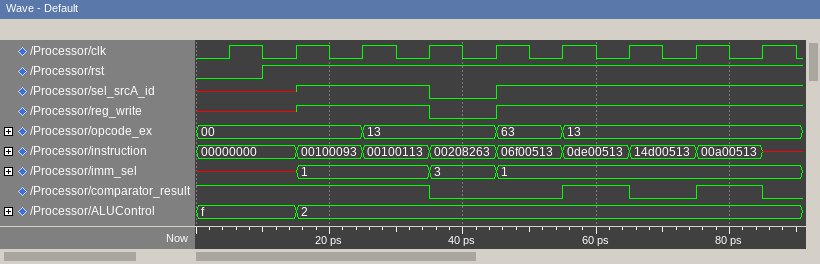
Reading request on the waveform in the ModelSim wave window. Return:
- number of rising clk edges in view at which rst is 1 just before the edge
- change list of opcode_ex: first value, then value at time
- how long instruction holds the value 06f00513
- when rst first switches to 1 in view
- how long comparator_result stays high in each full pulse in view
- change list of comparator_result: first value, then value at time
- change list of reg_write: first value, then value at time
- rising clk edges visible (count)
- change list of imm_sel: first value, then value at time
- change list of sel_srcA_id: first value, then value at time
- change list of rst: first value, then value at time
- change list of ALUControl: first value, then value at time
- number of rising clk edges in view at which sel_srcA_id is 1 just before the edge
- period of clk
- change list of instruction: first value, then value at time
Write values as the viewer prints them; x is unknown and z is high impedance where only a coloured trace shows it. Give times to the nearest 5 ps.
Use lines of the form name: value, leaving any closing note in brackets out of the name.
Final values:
number of rising clk edges in view at which rst is 1 just before the edge: 8
change list of opcode_ex: first value, then value at time: 00, 13 at 25 ps, 63 at 45 ps, 13 at 55 ps
how long instruction holds the value 06f00513: 10 ps
when rst first switches to 1 in view: 10 ps
how long comparator_result stays high in each full pulse in view: 10 ps, 10 ps
change list of comparator_result: first value, then value at time: 1, 0 at 35 ps, 1 at 55 ps, 0 at 65 ps, 1 at 75 ps, 0 at 85 ps
change list of reg_write: first value, then value at time: x, 1 at 15 ps, 0 at 35 ps, 1 at 45 ps
rising clk edges visible: 9
change list of imm_sel: first value, then value at time: x, 1 at 15 ps, 3 at 35 ps, 1 at 45 ps
change list of sel_srcA_id: first value, then value at time: x, 1 at 15 ps, 0 at 35 ps, 1 at 45 ps
change list of rst: first value, then value at time: 0, 1 at 10 ps
change list of ALUControl: first value, then value at time: f, 2 at 15 ps
number of rising clk edges in view at which sel_srcA_id is 1 just before the edge: 6
period of clk: 10 ps
change list of instruction: first value, then value at time: 00000000, 00100093 at 15 ps, 00100113 at 25 ps, 00208263 at 35 ps, 06f00513 at 45 ps, 0de00513 at 55 ps, 14d00513 at 65 ps, 00a00513 at 75 ps, x at 85 ps
